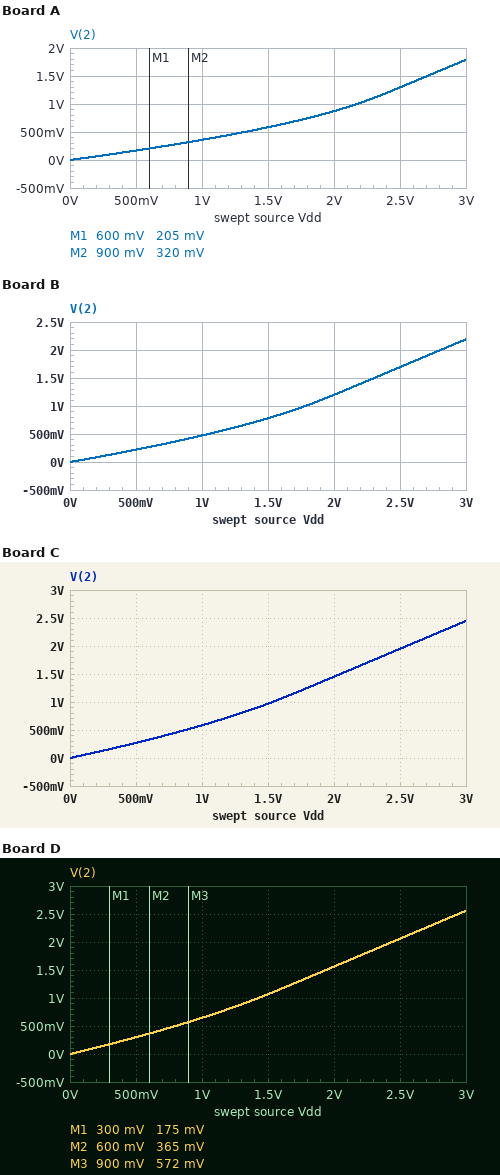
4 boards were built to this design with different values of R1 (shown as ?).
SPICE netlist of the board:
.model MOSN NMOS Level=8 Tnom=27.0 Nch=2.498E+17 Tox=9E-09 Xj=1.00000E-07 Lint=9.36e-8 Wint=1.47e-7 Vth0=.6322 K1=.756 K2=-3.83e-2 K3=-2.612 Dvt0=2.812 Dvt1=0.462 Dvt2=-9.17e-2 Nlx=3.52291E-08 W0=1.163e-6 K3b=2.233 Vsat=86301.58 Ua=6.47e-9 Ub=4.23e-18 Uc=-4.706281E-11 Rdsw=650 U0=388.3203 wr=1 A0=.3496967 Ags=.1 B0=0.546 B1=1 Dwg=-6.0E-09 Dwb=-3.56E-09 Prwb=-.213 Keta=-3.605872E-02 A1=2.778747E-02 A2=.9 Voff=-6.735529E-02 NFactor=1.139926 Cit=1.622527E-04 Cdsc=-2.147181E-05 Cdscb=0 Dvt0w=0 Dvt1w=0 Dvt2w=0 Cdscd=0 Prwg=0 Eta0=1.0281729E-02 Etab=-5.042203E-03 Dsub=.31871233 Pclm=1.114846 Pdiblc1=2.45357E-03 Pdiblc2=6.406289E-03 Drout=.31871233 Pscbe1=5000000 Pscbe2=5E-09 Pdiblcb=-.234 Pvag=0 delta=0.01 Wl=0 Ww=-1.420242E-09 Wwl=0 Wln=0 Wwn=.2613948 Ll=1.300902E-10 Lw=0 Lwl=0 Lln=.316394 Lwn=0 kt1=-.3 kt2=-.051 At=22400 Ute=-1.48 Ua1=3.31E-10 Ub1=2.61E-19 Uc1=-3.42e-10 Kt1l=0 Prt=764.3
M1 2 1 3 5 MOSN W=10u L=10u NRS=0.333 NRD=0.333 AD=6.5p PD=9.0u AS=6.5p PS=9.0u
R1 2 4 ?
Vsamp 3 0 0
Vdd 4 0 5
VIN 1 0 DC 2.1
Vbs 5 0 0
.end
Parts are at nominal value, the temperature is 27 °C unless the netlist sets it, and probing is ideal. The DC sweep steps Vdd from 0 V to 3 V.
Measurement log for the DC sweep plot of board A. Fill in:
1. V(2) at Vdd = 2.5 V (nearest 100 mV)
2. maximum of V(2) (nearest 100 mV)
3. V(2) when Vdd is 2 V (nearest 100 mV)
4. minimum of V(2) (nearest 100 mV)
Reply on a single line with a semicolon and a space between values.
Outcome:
1.3 V; 1.8 V; 900 mV; 0 V
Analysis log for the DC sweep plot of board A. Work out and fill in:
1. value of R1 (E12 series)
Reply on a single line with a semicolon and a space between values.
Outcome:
33 kΩ
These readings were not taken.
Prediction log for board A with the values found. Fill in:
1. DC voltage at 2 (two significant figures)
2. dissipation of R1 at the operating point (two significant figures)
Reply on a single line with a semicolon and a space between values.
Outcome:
3.8 V; 45 µW
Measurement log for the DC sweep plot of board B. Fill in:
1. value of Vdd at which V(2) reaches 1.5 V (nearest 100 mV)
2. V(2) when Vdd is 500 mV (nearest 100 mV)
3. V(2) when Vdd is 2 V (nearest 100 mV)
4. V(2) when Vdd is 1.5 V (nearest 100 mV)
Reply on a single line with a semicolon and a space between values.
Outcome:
2.3 V; 200 mV; 1.2 V; 800 mV
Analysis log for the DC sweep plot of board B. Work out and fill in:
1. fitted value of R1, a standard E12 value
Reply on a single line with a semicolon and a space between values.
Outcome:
22 kΩ
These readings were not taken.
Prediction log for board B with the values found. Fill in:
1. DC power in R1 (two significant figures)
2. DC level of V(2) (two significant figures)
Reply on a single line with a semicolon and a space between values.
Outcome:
30 µW; 4.2 V
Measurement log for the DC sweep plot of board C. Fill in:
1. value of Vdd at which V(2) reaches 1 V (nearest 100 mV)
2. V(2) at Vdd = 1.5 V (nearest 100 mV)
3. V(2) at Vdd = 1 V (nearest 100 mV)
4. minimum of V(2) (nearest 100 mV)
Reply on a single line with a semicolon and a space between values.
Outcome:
1.5 V; 1.0 V; 600 mV; 0 V
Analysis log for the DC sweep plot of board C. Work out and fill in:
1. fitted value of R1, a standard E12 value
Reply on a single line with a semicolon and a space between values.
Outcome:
15 kΩ
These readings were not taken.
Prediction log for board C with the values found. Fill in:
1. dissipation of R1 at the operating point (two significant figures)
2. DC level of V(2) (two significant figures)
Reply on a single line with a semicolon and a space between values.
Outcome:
21 µW; 4.4 V
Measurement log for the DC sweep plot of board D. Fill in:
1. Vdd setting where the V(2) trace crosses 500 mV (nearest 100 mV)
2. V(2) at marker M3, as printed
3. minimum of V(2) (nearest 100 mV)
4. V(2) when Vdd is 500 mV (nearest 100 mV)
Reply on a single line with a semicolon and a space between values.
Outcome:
800 mV; 572 mV; 0 V; 300 mV
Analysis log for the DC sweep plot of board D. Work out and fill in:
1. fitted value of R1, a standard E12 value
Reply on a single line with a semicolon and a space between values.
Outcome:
12 kΩ
